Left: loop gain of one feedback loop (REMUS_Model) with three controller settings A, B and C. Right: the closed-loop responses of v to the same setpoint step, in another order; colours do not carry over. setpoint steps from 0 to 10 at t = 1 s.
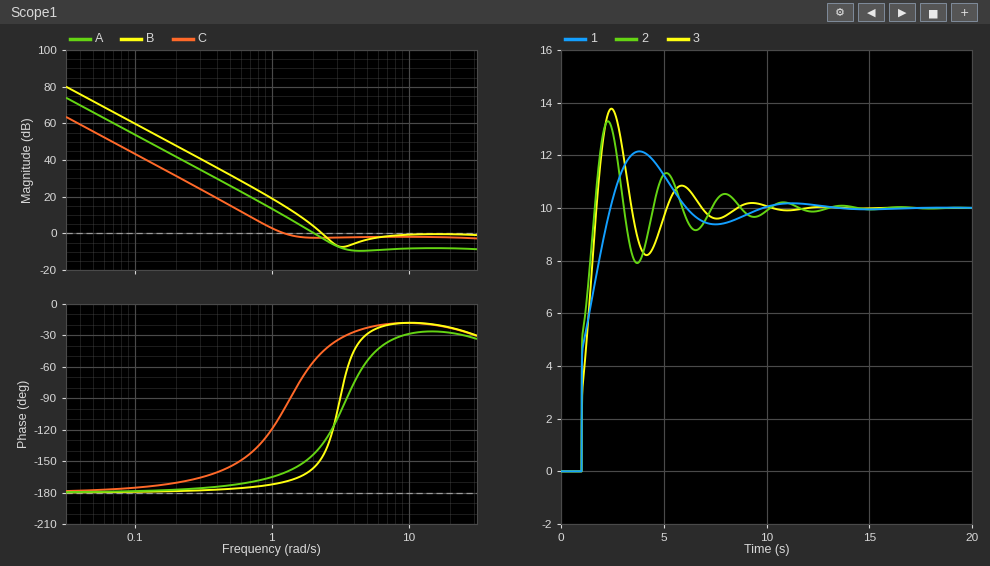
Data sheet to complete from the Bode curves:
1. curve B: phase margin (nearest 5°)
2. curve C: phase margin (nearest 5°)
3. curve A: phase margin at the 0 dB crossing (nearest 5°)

35°
80°
35°
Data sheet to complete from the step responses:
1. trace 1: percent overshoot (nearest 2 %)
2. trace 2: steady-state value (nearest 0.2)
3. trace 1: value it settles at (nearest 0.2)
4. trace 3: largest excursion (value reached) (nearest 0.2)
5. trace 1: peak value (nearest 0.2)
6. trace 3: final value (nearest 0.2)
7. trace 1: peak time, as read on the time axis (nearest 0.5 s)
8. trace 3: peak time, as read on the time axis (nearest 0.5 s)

22 %
10.0
10.0
13.8
12.2
10.0
4.0 s
2.5 s
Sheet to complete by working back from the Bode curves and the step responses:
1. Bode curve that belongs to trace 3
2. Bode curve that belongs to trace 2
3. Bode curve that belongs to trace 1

A
B
C
